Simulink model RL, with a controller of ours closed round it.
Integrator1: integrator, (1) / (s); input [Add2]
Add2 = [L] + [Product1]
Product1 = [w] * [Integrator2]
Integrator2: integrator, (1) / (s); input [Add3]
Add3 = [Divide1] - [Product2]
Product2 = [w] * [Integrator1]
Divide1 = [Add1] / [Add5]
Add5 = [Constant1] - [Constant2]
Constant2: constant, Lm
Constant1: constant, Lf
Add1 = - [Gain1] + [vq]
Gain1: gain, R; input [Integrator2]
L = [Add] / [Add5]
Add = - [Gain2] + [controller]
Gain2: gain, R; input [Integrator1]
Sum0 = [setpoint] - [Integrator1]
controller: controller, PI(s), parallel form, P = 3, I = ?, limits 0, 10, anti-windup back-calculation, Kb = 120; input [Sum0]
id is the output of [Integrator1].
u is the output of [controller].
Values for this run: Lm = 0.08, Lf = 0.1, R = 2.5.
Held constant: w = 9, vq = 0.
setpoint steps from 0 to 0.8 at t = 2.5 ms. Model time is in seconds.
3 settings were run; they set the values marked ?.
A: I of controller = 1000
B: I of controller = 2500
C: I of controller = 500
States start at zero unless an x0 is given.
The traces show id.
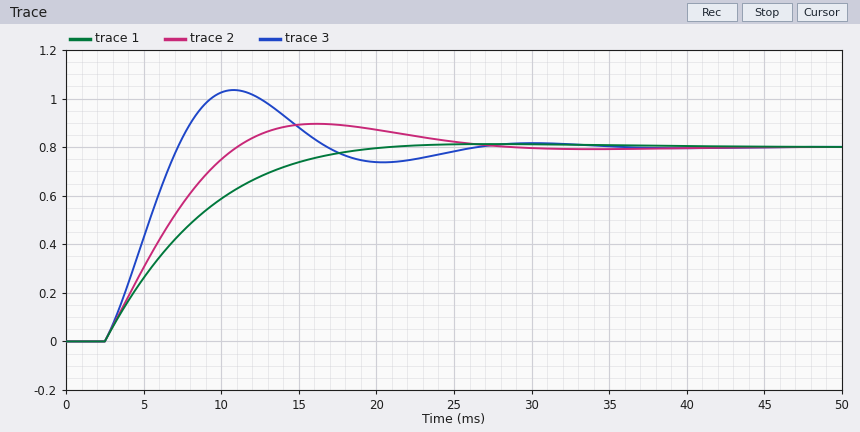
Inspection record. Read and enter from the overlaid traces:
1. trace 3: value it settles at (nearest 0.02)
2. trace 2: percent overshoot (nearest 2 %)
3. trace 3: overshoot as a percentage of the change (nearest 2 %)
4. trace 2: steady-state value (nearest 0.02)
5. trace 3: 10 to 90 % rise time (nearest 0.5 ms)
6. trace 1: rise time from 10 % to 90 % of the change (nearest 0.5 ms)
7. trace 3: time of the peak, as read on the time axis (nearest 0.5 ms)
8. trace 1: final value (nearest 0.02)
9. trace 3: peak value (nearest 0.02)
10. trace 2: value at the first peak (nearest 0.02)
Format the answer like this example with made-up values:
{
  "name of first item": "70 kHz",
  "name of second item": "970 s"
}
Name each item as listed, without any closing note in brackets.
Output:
{
  "trace 3: value it settles at": "0.80",
  "trace 2: percent overshoot": "12 %",
  "trace 3: overshoot as a percentage of the change": "30 %",
  "trace 2: steady-state value": "0.80",
  "trace 3: 10 to 90 % rise time": "3.5 ms",
  "trace 1: rise time from 10 % to 90 % of the change": "11.0 ms",
  "trace 3: time of the peak, as read on the time axis": "11.0 ms",
  "trace 1: final value": "0.80",
  "trace 3: peak value": "1.04",
  "trace 2: value at the first peak": "0.90"
}
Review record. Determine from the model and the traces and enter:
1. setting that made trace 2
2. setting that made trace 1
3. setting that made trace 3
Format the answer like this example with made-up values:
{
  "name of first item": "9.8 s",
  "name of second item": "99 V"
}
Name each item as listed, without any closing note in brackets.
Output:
{
  "setting that made trace 2": "A",
  "setting that made trace 1": "C",
  "setting that made trace 3": "B"
}
